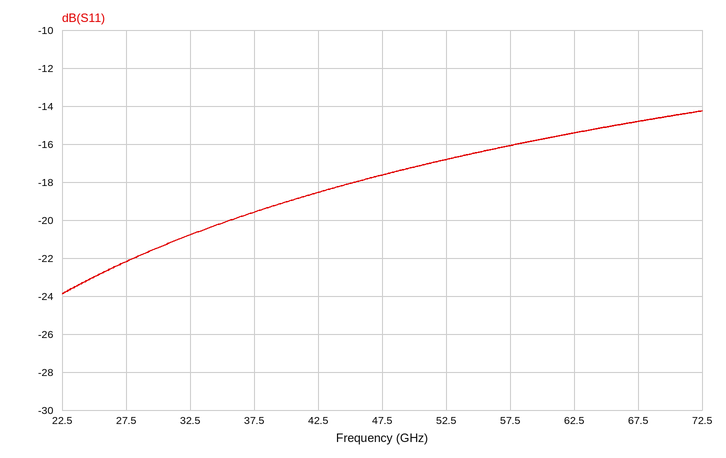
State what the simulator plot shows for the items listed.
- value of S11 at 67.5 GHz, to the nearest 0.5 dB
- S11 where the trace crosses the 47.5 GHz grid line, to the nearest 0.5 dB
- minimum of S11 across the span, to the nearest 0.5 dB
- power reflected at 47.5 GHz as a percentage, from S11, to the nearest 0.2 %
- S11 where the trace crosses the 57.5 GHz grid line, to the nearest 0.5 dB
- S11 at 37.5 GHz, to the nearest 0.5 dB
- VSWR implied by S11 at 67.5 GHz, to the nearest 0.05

-15.0 dB
-17.5 dB
-24.0 dB
1.8 %
-16.0 dB
-19.5 dB
1.45
